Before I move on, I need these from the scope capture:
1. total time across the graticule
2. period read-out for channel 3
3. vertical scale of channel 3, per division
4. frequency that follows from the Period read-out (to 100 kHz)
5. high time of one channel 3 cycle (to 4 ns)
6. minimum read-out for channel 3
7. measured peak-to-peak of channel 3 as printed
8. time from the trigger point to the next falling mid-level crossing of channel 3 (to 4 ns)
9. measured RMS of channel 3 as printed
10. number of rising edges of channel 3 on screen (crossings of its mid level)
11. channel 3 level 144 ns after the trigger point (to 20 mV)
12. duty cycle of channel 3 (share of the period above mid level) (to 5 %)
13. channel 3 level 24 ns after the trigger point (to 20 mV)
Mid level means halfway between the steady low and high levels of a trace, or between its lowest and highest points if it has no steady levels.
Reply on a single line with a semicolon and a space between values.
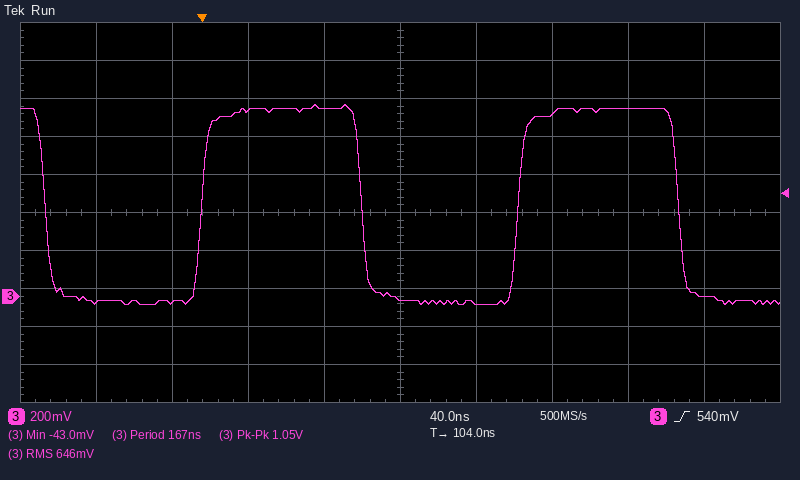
400 ns; 167 ns; 200 mV; 6.0 MHz; 84 ns; -43.0 mV; 1.05 V; 84 ns; 646 mV; 2; -40 mV; 50 %; 980 mV
